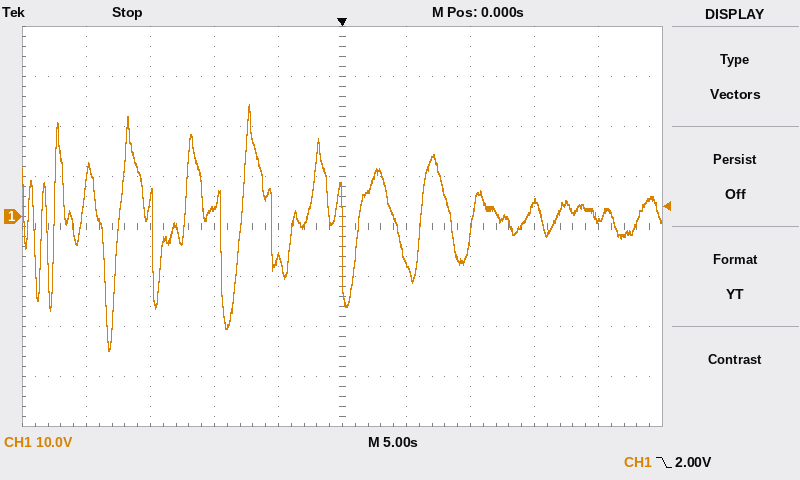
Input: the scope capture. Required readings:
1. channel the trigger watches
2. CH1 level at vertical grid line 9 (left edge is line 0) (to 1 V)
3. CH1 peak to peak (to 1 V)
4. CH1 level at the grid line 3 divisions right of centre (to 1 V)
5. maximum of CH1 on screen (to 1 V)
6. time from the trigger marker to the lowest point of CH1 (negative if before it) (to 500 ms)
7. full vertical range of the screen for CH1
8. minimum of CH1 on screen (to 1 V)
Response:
CH1
0 V
49 V
3 V
22 V
-18.0 s
80 V
-27 V
